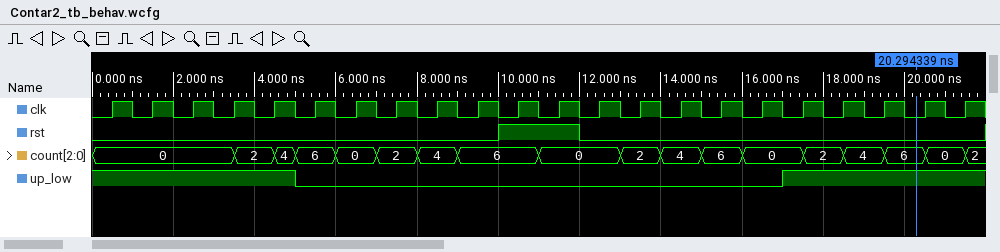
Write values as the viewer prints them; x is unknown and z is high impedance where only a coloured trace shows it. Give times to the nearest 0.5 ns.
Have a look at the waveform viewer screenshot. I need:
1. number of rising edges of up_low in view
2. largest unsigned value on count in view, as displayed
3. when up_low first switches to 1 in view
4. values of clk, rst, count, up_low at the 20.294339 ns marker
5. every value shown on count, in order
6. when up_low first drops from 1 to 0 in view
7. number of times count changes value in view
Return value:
1
6
17 ns
clk=0, rst=0, count=6, up_low=1
0, 2, 4, 6, 0, 2, 4, 6, 0, 2, 4, 6, 0, 2, 4, 6, 0, 2
5 ns
17
